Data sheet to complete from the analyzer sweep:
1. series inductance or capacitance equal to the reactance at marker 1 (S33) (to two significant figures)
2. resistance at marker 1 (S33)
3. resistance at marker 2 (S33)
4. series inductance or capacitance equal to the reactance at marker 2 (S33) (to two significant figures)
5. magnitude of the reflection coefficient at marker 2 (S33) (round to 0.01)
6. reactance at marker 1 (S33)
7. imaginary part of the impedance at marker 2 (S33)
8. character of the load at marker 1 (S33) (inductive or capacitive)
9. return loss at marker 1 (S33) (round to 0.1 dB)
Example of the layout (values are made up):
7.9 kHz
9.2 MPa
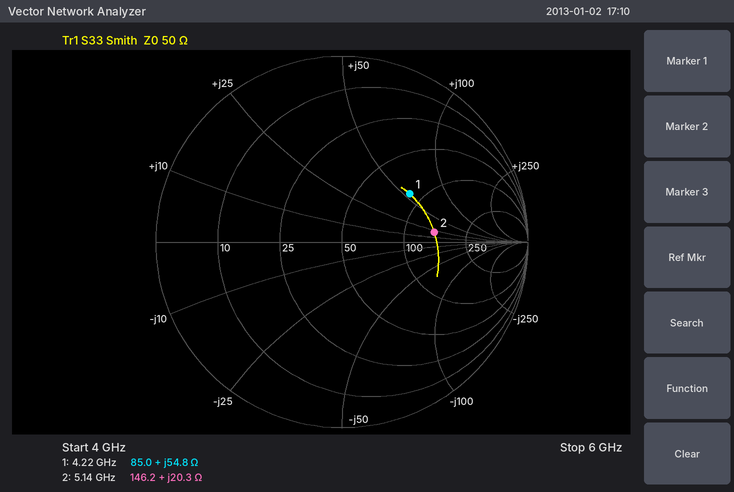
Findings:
2.1 nH
85.0 Ω
146.2 Ω
630 pH
0.50
+54.8 Ω
+20.3 Ω
inductive
7.0 dB
